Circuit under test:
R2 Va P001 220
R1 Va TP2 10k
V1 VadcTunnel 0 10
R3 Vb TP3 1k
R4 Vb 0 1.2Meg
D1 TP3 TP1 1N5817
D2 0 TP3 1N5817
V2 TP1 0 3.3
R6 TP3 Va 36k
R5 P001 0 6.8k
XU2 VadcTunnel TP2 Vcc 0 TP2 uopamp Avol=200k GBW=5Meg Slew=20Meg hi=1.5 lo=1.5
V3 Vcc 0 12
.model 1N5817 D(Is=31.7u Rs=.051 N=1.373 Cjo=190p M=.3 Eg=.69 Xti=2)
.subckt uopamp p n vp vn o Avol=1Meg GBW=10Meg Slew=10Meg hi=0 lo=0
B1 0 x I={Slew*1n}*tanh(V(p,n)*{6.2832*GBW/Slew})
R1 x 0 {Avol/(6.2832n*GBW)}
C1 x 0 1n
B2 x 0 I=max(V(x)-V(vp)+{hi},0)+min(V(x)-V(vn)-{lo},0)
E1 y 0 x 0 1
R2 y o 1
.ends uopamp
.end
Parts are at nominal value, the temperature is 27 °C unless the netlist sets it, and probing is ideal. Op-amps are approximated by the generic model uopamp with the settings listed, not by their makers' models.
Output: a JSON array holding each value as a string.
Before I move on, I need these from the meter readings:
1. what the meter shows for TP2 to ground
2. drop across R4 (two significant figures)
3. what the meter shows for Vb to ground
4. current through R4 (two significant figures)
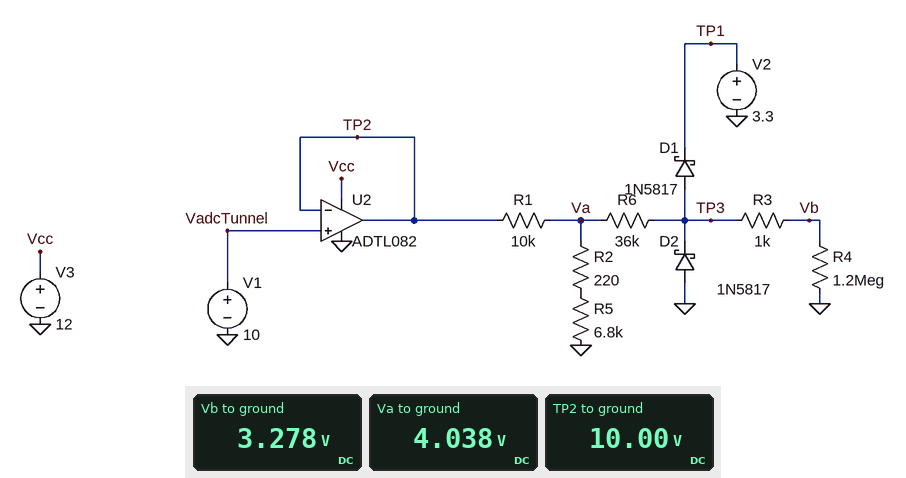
["10.00 V", "3.3 V", "3.278 V", "2.7 µA"]
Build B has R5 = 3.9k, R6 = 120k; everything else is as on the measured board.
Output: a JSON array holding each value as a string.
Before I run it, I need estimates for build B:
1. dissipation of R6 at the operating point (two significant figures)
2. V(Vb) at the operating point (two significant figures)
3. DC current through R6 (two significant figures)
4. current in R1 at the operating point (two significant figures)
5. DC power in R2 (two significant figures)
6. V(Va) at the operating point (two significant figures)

["590 nW", "2.6 V", "2.2 µA", "710 µA", "110 µW", "2.9 V"]
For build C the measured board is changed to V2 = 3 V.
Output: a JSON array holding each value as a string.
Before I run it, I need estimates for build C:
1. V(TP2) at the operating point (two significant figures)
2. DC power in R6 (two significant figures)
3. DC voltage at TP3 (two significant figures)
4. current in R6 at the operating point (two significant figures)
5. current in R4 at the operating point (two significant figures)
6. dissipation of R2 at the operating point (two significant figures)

["10 V", "29 µW", "3.0 V", "28 µA", "2.5 µA", "72 µW"]
